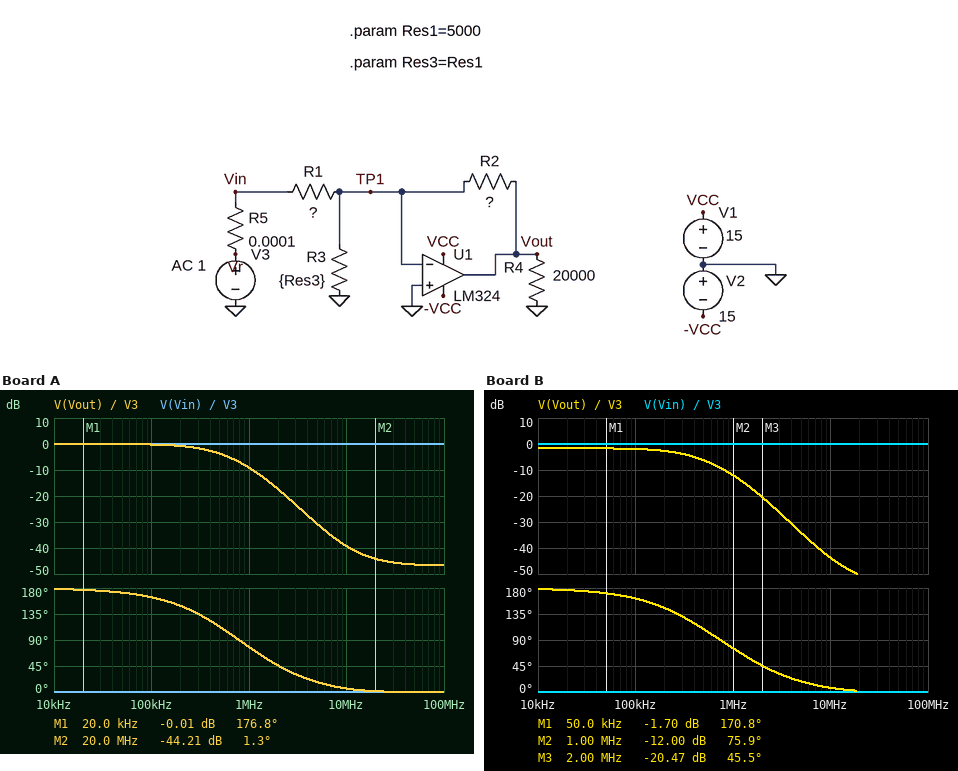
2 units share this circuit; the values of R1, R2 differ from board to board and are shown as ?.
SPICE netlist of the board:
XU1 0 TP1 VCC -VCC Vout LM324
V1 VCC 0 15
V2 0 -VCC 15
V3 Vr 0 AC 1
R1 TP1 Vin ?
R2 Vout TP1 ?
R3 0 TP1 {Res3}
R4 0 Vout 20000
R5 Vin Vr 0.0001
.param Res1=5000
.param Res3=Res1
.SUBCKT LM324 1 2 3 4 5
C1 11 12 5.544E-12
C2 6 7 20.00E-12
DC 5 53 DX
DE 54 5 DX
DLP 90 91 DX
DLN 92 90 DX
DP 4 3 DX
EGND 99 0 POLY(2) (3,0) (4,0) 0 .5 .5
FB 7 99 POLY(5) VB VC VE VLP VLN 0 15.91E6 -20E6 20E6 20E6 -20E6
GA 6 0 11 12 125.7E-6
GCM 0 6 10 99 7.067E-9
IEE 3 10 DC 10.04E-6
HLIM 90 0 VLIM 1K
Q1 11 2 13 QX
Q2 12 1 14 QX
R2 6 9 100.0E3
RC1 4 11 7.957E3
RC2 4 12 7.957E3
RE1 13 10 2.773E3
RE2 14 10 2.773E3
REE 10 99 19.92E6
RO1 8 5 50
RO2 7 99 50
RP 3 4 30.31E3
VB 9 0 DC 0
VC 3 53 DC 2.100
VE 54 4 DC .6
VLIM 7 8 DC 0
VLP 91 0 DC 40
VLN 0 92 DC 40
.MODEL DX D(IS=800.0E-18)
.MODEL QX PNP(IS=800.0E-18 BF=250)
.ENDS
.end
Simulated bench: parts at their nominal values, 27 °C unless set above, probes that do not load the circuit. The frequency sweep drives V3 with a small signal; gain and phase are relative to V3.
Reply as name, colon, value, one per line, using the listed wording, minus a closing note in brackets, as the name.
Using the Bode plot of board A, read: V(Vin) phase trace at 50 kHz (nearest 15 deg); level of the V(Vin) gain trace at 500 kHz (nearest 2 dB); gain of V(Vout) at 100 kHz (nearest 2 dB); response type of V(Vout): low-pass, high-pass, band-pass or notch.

V(Vin) phase trace at 50 kHz: 0 deg
level of the V(Vin) gain trace at 500 kHz: 0 dB
gain of V(Vout) at 100 kHz: 0 dB
response type of V(Vout): low-pass, high-pass, band-pass or notch: low-pass
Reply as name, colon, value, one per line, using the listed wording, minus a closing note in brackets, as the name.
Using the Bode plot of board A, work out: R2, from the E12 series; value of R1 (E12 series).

R2, from the E12 series: 3.9 kΩ
value of R1: 3.9 kΩ
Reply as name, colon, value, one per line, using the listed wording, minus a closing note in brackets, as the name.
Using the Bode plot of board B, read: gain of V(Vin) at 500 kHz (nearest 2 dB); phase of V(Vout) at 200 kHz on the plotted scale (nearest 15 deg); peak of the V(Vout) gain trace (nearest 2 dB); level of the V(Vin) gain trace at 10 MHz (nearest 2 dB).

gain of V(Vin) at 500 kHz: 0 dB
phase of V(Vout) at 200 kHz on the plotted scale: 150 deg
peak of the V(Vout) gain trace: -2 dB
level of the V(Vin) gain trace at 10 MHz: 0 dB
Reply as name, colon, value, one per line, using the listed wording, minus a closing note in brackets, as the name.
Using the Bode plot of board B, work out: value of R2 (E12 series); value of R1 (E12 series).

value of R2: 6.8 kΩ
value of R1: 8.2 kΩ
